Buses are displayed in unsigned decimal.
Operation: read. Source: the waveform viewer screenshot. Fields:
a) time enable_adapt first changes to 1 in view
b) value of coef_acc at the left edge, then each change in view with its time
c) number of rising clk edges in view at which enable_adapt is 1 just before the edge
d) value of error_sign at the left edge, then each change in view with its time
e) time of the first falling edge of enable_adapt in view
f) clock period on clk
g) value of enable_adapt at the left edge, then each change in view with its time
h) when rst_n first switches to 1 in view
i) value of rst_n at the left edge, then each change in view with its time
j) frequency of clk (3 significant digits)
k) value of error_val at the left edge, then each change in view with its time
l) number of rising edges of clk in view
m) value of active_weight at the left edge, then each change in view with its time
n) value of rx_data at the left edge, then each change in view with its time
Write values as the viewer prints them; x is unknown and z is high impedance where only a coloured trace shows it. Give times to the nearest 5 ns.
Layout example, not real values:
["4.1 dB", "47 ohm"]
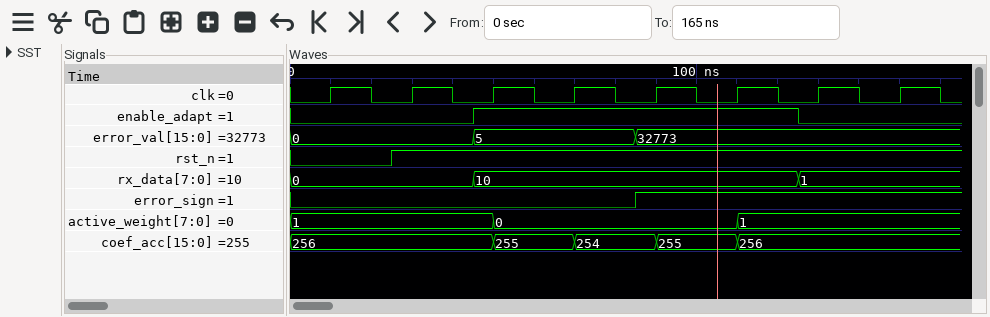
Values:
["45 ns", "256, 255 at 50 ns, 254 at 70 ns, 255 at 90 ns, 256 at 110 ns", "4", "0, 1 at 85 ns", "125 ns", "20 ns", "0, 1 at 45 ns, 0 at 125 ns", "25 ns", "0, 1 at 25 ns", "50.0 MHz", "0, 5 at 45 ns, 32773 at 85 ns", "8", "1, 0 at 50 ns, 1 at 110 ns", "0, 10 at 45 ns, 1 at 125 ns"]
